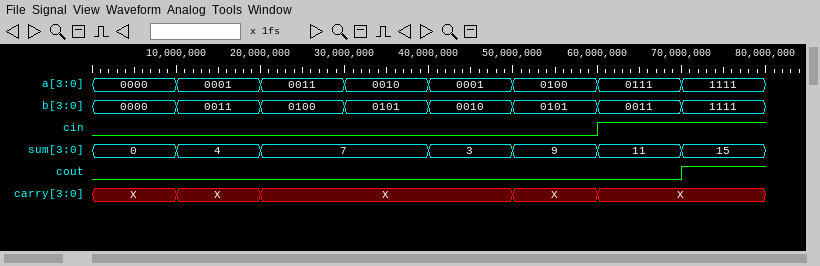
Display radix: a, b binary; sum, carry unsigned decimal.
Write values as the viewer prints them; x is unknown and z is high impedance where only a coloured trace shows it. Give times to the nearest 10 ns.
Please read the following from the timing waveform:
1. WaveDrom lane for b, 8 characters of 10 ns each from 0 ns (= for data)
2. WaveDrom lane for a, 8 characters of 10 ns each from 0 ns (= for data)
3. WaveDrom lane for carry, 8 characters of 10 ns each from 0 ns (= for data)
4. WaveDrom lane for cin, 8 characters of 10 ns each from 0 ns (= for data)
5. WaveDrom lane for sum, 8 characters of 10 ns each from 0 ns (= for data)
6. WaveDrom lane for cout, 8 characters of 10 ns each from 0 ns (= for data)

{name: 'b', wave: '========', data: '0000 0011 0100 0101 0010 0101 0011 1111'}
{name: 'a', wave: '========', data: '0000 0001 0011 0010 0001 0100 0111 1111'}
{name: 'carry', wave: '===..==.', data: 'X X X X X'}
{name: 'cin', wave: '0.....1.'}
{name: 'sum', wave: '===.====', data: '0 4 7 3 9 11 15'}
{name: 'cout', wave: '0......1'}
